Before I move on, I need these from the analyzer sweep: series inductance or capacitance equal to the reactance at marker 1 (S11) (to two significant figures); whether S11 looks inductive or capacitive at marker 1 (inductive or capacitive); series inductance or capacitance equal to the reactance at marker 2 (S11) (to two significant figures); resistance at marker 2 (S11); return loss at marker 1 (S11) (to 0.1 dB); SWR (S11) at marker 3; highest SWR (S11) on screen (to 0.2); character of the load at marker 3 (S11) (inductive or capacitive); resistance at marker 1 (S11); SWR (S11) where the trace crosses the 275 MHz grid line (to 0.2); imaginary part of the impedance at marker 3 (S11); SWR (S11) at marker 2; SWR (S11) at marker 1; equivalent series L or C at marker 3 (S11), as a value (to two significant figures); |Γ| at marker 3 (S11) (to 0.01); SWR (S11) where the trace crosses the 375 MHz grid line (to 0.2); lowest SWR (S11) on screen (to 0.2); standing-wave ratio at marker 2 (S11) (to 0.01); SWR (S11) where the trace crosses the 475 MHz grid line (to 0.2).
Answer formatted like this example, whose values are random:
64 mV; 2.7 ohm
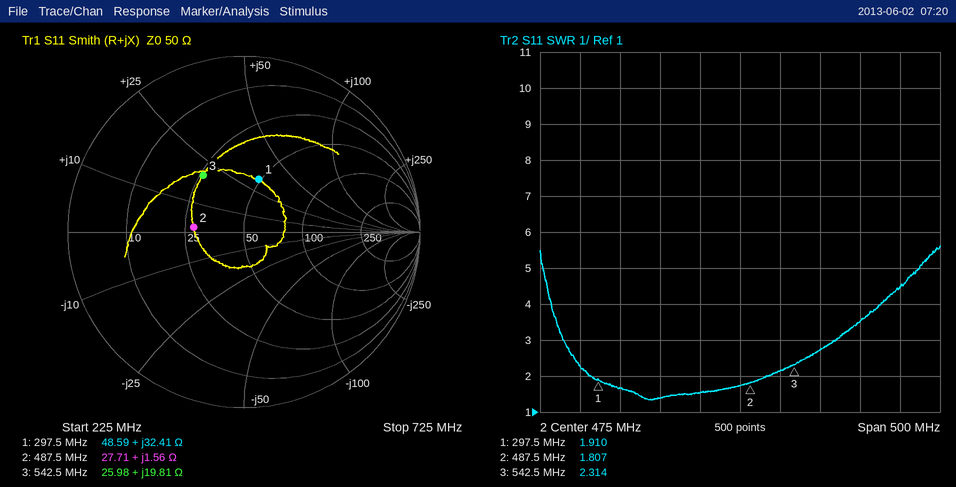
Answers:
17 nH; inductive; 510 pH; 27.71 Ω; 10.1 dB; 2.314; 5.6; inductive; 48.59 Ω; 2.2; +19.81 Ω; 1.807; 1.910; 5.8 nH; 0.40; 1.4; 1.4; 1.81; 1.8
